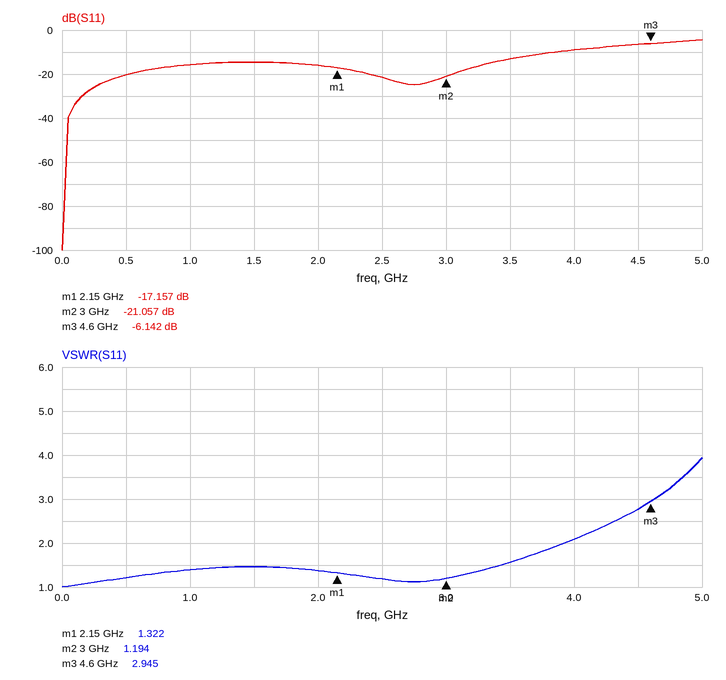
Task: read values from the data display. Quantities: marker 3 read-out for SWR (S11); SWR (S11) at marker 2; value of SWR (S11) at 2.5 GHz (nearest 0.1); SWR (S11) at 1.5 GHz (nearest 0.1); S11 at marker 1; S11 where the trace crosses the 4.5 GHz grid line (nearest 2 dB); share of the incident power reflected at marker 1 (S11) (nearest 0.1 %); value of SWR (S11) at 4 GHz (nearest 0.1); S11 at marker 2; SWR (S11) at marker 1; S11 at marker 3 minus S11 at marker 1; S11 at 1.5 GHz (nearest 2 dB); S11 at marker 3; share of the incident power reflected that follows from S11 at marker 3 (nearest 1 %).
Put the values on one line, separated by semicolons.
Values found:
2.945; 1.194; 1.2; 1.5; -17.157 dB; -6 dB; 1.9 %; 2.1; -21.057 dB; 1.322; 11.015 dB; -14 dB; -6.142 dB; 24 %
